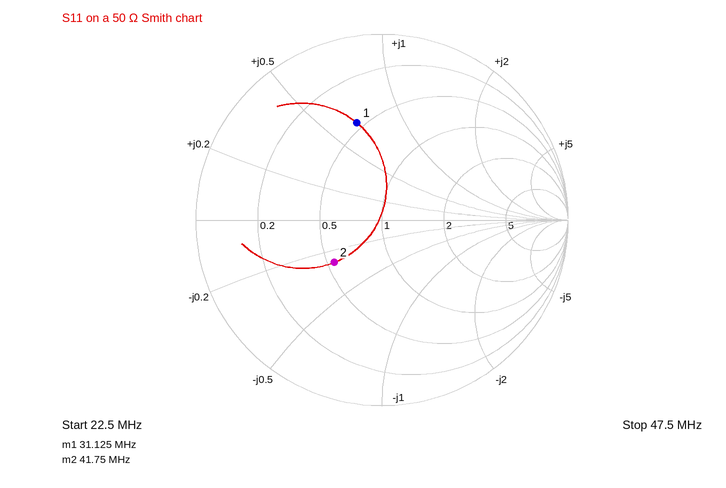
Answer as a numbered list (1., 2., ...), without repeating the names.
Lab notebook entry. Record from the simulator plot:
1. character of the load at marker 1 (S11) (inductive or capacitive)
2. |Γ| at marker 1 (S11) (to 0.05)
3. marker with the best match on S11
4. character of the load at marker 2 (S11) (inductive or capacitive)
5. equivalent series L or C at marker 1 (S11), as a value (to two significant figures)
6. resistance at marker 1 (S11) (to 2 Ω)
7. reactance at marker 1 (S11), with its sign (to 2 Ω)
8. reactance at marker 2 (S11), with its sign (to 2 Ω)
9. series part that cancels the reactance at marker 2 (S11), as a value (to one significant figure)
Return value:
1. inductive
2. 0.55
3. marker 2
4. capacitive
5. 170 nH
6. 22 Ω
7. +34 Ω
8. -14 Ω
9. 50 nH
